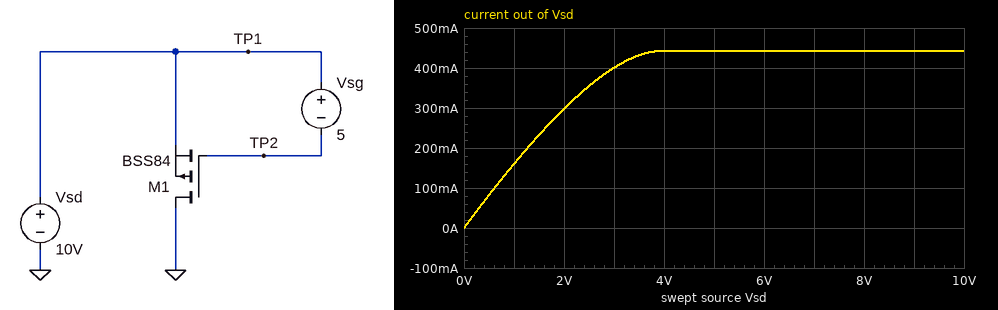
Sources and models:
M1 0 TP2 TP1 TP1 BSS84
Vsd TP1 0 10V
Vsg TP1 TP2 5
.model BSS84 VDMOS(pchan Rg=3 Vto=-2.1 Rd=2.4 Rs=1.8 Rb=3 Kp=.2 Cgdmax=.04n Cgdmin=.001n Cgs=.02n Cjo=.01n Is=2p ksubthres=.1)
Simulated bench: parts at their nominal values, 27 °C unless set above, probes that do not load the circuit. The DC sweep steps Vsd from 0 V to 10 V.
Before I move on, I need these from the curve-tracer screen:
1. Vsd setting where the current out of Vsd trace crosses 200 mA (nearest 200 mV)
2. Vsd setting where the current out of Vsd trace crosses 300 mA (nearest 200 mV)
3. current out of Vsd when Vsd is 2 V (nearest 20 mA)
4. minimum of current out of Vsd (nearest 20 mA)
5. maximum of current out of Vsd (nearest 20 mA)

1.2 V
2.0 V
300 mA
0 A
440 mA
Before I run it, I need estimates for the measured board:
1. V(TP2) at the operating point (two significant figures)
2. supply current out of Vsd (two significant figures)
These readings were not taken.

5.0 V
440 mA
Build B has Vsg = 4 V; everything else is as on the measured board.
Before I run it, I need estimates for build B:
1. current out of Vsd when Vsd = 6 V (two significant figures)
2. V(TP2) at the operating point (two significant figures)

220 mA
6.0 V
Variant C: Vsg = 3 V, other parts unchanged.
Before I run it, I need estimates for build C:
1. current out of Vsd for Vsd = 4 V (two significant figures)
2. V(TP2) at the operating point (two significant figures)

62 mA
7.0 V
